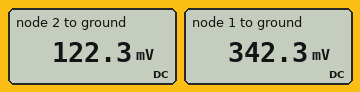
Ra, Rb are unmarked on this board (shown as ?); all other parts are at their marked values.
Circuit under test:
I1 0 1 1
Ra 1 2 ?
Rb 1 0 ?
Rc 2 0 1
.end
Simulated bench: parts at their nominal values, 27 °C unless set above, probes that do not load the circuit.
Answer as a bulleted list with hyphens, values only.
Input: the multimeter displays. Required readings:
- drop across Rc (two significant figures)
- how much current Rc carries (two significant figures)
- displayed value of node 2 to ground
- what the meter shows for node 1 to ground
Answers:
- 120 mV
- 120 mA
- 122.3 mV
- 342.3 mV
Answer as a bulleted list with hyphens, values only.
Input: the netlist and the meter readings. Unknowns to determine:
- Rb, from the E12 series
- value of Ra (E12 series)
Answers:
- 0.39 Ω
- 1.8 Ω
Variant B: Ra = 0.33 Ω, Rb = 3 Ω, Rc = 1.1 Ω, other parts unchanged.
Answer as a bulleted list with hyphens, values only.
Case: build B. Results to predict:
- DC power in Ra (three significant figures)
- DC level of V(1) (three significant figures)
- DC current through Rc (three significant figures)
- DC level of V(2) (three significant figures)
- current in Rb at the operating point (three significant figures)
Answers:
- 151 mW
- 968 mV
- 677 mA
- 745 mV
- 323 mA
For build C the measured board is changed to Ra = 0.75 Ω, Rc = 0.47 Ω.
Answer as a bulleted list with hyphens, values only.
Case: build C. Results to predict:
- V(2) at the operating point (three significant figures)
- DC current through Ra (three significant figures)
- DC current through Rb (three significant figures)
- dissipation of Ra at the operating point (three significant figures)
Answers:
- 114 mV
- 242 mA
- 758 mA
- 44.0 mW
